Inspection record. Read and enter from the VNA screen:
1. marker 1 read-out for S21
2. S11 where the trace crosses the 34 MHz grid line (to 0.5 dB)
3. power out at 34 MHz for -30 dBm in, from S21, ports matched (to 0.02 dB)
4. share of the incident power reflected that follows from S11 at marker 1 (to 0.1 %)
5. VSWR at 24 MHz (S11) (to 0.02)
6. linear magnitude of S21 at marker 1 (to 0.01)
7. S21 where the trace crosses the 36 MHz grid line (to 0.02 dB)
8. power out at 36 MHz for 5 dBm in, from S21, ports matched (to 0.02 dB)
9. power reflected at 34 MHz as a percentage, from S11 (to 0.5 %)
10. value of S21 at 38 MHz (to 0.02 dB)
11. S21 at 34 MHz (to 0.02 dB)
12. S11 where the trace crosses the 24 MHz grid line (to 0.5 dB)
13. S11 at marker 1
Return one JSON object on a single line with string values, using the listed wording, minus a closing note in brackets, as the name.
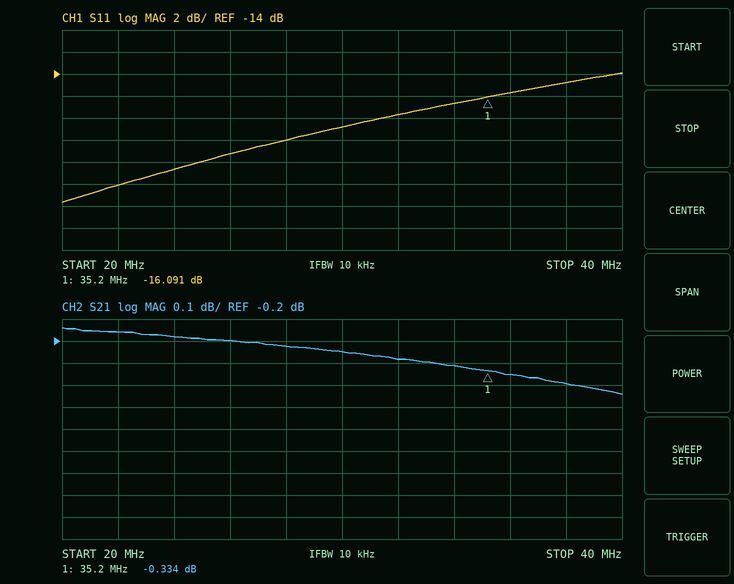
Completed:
{"marker 1 read-out for S21": "-0.334 dB", "S11 where the trace crosses the 34 MHz grid line": "-16.5 dB", "power out at 34 MHz for -30 dBm in, from S21, ports matched": "-30.32 dBm", "share of the incident power reflected that follows from S11 at marker 1": "2.5 %", "VSWR at 24 MHz (S11)": "1.16", "linear magnitude of S21 at marker 1": "0.96", "S21 where the trace crosses the 36 MHz grid line": "-0.36 dB", "power out at 36 MHz for 5 dBm in, from S21, ports matched": "4.64 dBm", "power reflected at 34 MHz as a percentage, from S11": "2.0 %", "value of S21 at 38 MHz": "-0.40 dB", "S21 at 34 MHz": "-0.32 dB", "S11 where the trace crosses the 24 MHz grid line": "-22.5 dB", "S11 at marker 1": "-16.091 dB"}
